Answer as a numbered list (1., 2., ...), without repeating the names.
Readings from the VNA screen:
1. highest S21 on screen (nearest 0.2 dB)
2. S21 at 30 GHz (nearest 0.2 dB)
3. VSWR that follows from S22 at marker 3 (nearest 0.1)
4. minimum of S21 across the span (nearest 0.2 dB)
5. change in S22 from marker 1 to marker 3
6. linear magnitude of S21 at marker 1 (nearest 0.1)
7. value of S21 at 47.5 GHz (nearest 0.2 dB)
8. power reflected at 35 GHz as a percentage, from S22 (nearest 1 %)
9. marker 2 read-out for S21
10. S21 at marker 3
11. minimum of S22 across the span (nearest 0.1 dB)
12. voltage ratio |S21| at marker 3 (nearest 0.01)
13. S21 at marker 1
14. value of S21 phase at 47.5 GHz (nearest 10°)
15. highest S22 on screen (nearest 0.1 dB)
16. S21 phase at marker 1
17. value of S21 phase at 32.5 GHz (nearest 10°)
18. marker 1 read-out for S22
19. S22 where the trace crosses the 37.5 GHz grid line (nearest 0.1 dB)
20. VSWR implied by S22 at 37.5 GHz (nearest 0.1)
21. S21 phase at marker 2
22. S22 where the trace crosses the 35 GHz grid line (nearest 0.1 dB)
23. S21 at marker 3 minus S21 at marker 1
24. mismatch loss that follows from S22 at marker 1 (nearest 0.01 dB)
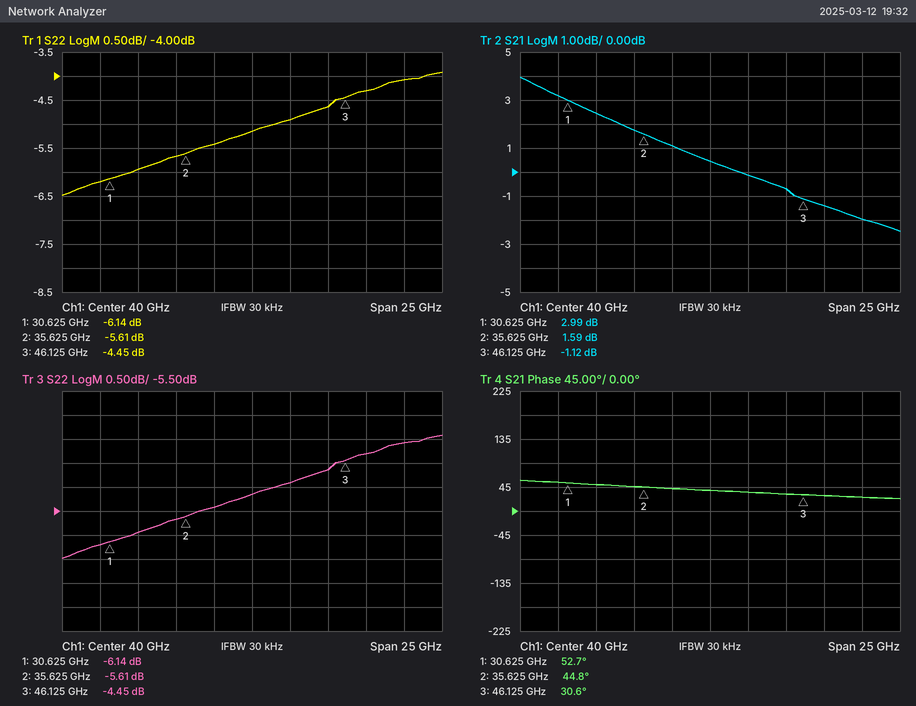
1. 4.0 dB
2. 3.2 dB
3. 4.0
4. -2.4 dB
5. 1.69 dB
6. 1.4
7. -1.4 dB
8. 27 %
9. 1.59 dB
10. -1.12 dB
11. -6.5 dB
12. 0.88
13. 2.99 dB
14. 30°
15. -3.9 dB
16. 52.7°
17. 50°
18. -6.14 dB
19. -5.4 dB
20. 3.3
21. 44.8°
22. -5.7 dB
23. -4.11 dB
24. 1.21 dB
